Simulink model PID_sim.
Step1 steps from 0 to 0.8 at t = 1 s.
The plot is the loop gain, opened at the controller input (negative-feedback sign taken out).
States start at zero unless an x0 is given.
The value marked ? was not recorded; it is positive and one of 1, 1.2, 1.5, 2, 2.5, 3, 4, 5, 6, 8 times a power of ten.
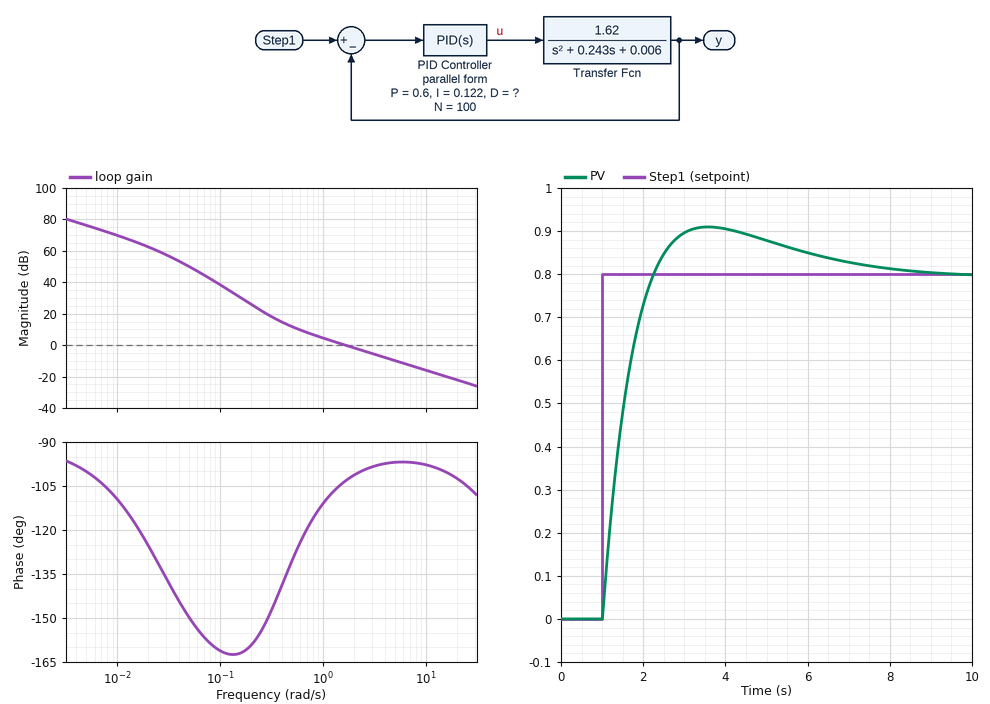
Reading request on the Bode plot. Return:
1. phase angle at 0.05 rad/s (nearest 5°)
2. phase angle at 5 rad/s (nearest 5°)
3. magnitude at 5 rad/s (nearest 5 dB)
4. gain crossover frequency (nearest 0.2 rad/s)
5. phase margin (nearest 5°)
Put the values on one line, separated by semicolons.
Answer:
-150°; -95°; -10 dB; 1.6 rad/s; 75°
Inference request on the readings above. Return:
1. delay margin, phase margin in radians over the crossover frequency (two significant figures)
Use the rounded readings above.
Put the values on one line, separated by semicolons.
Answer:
0.82 s
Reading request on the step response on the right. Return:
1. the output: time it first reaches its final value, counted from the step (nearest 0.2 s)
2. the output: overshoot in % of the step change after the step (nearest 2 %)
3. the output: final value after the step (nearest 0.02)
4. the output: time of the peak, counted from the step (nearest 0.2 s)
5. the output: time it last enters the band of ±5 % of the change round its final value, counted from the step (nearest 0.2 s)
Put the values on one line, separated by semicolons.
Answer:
1.2 s; 14 %; 0.80; 2.6 s; 5.4 s
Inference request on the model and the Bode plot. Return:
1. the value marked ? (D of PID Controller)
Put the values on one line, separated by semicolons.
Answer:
1
